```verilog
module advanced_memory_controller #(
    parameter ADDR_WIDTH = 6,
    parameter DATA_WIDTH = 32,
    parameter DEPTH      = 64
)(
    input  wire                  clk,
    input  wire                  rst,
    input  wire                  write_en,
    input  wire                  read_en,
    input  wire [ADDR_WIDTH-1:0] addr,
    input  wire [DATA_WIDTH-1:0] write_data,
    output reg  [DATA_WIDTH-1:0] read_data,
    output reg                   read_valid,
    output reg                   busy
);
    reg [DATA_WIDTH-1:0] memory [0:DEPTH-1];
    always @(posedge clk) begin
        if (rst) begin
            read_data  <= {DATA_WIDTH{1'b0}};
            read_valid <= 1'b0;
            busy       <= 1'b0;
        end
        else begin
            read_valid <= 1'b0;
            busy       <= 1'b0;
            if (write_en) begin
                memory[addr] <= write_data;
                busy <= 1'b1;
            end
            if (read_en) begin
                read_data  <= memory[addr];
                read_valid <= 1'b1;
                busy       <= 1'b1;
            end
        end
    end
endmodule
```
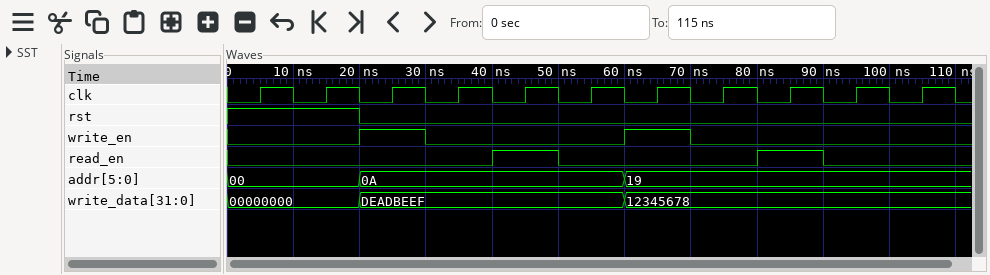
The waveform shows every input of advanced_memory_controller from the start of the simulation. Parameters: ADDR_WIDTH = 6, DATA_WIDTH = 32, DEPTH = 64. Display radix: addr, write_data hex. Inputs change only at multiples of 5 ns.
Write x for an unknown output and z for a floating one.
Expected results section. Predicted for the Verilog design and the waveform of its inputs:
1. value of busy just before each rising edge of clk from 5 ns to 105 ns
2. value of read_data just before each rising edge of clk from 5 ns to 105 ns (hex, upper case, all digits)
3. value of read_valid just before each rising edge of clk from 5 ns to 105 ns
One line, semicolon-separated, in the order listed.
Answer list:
x 0 0 1 0 1 0 1 0 1 0; x, 00000000, 00000000, 00000000, 00000000, DEADBEEF, DEADBEEF, DEADBEEF, DEADBEEF, 12345678, 12345678; x 0 0 0 0 1 0 0 0 1 0
